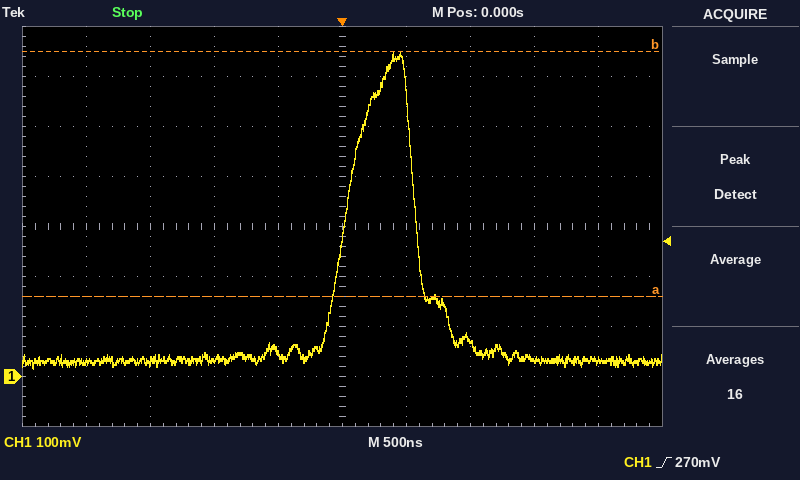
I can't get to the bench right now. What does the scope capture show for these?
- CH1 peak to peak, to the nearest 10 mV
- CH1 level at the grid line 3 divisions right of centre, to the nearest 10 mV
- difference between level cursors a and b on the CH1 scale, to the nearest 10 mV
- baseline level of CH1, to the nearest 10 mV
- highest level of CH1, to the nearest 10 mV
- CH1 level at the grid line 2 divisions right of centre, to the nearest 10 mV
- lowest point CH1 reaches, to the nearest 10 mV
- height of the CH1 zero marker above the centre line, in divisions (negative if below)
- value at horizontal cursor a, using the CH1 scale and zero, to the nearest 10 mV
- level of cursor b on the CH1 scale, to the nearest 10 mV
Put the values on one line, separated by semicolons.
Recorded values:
630 mV; 30 mV; 490 mV; 30 mV; 650 mV; 70 mV; 20 mV; -3.0 div; 160 mV; 650 mV
